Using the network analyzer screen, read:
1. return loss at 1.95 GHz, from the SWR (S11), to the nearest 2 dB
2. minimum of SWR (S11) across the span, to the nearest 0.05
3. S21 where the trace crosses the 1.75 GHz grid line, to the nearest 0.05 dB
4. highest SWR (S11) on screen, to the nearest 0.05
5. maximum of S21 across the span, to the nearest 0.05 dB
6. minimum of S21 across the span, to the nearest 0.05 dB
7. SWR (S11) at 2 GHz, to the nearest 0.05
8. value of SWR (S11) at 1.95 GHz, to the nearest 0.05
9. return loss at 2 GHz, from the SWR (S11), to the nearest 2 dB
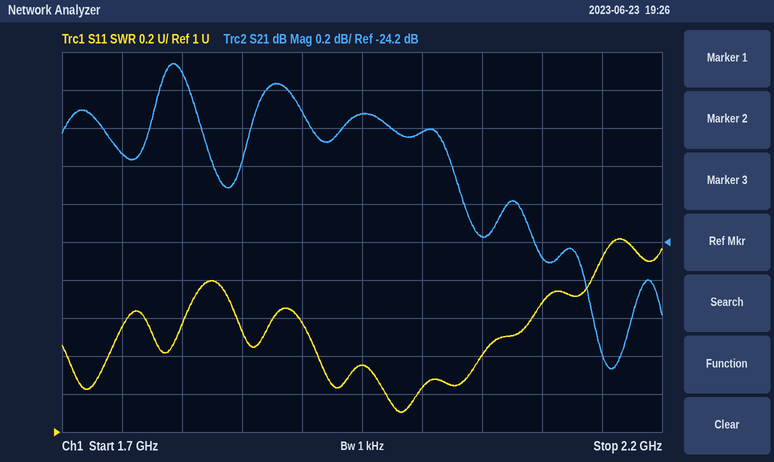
16 dB
1.10
-23.75 dB
2.00
-23.25 dB
-24.85 dB
1.25
1.35
20 dB
